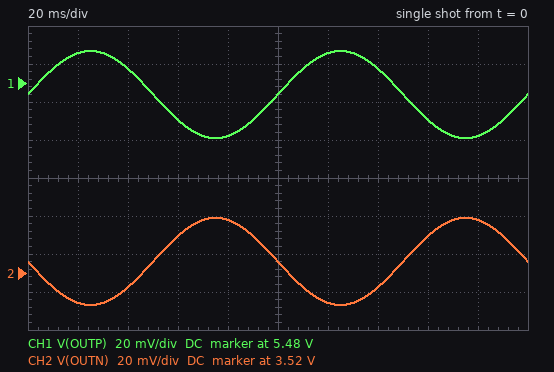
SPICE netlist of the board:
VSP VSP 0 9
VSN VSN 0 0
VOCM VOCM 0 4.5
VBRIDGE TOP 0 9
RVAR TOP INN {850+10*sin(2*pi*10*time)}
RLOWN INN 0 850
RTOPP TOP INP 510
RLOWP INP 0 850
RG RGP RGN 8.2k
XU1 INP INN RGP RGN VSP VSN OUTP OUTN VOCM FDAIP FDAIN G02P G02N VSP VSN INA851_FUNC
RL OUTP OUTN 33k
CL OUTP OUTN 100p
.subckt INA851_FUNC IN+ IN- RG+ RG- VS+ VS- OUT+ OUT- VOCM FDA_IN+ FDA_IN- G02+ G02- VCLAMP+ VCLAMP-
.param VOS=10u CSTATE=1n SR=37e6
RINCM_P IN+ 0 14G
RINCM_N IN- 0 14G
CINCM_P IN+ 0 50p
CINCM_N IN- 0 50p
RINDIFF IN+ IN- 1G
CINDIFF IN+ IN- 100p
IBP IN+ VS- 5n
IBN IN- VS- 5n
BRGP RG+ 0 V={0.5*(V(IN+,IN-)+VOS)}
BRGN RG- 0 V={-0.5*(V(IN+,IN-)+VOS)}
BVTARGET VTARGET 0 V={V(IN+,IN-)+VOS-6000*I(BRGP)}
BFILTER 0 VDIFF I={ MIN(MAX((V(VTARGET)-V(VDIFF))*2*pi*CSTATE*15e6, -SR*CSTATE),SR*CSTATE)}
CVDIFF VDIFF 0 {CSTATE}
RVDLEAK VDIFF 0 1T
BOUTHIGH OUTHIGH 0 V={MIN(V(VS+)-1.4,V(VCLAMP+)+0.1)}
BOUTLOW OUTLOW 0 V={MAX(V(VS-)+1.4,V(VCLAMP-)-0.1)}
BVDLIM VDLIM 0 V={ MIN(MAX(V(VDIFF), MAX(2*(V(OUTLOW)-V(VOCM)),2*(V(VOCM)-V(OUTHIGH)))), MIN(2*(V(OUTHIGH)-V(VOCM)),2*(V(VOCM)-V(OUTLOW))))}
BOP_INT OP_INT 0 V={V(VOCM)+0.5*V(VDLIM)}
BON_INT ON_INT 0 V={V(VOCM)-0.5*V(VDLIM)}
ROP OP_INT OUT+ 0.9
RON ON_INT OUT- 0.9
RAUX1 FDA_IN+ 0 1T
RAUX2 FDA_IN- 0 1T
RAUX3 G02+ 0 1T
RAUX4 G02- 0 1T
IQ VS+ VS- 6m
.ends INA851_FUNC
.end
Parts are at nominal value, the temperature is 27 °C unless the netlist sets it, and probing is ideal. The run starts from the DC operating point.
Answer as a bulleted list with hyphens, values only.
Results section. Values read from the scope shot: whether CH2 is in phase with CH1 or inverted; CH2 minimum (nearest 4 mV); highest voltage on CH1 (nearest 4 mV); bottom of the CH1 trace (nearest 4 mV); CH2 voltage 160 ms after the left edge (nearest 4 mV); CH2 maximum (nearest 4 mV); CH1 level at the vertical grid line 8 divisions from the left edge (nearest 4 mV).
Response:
- inverted
- 3.504 V
- 5.496 V
- 5.452 V
- 3.540 V
- 3.548 V
- 5.460 V
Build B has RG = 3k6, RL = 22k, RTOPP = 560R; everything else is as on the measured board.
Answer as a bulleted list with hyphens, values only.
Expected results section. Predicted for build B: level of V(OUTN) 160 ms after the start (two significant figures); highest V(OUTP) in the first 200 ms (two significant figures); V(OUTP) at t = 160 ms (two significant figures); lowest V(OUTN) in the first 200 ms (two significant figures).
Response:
- 3.3 V
- 5.8 V
- 5.7 V
- 3.2 V
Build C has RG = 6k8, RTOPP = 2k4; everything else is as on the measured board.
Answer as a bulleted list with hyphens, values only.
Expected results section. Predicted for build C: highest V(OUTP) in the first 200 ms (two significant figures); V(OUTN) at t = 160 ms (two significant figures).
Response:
- 2.5 V
- 6.5 V
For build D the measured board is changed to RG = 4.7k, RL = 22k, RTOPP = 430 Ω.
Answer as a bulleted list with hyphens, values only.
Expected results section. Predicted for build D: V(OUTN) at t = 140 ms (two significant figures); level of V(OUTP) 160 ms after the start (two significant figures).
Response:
- 2.8 V
- 6.2 V
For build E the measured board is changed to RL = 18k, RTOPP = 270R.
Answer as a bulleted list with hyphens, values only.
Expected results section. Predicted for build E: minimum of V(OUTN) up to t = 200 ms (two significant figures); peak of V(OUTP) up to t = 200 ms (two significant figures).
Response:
- 2.5 V
- 6.5 V
